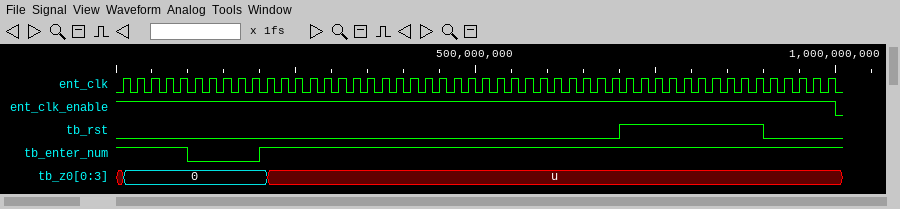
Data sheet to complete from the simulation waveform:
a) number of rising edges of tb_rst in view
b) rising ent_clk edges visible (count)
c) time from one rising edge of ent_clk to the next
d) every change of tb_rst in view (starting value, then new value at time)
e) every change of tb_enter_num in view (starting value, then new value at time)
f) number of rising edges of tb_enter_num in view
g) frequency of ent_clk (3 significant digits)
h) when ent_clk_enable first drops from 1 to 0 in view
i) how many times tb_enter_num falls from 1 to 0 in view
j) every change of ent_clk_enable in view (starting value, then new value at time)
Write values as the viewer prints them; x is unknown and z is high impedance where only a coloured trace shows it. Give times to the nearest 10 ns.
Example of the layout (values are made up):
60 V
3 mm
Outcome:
1
50
20 ns
0, 1 at 700 ns, 0 at 900 ns
1, 0 at 100 ns, 1 at 200 ns
1
50.0 MHz
1000 ns
1
1, 0 at 1000 ns
